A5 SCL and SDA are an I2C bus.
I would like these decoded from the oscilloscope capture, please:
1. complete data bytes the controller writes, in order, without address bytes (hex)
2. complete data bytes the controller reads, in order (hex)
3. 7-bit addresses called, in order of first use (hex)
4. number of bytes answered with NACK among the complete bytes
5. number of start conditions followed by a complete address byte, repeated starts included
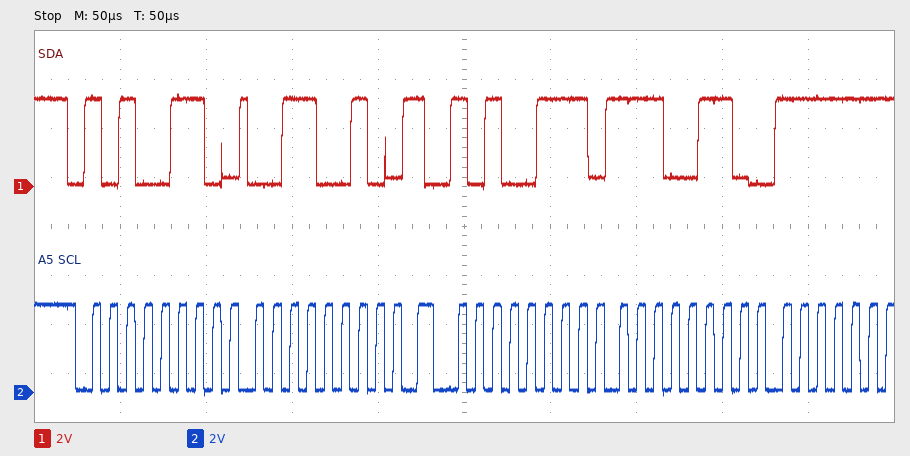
32
E6
0x53
0
2
